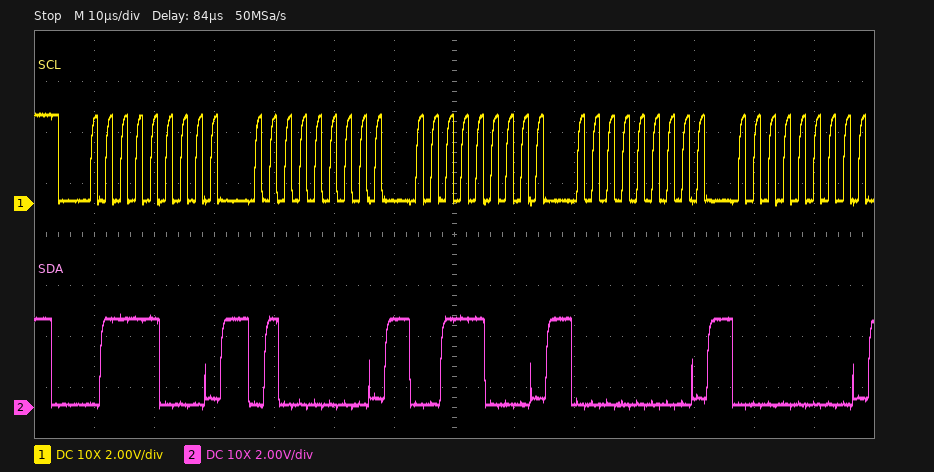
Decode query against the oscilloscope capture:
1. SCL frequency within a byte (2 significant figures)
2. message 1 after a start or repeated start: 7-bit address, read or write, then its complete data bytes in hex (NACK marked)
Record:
400 kHz
0x3C write: 40 38 00 00
